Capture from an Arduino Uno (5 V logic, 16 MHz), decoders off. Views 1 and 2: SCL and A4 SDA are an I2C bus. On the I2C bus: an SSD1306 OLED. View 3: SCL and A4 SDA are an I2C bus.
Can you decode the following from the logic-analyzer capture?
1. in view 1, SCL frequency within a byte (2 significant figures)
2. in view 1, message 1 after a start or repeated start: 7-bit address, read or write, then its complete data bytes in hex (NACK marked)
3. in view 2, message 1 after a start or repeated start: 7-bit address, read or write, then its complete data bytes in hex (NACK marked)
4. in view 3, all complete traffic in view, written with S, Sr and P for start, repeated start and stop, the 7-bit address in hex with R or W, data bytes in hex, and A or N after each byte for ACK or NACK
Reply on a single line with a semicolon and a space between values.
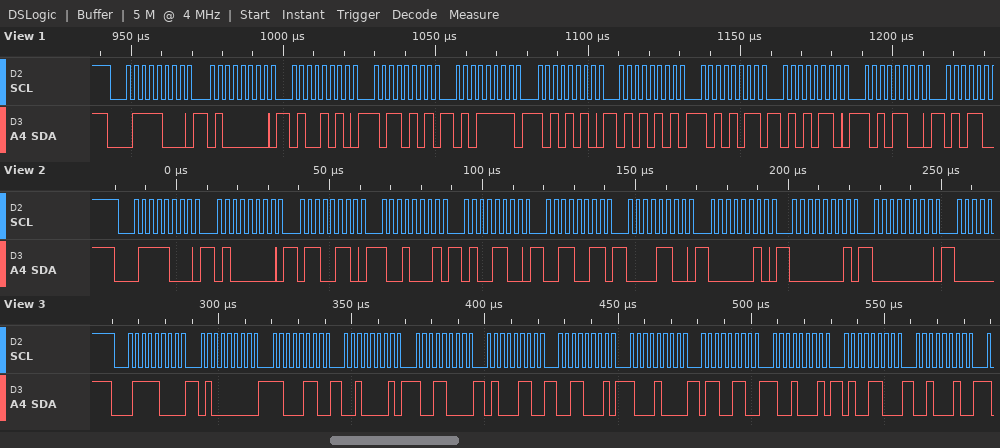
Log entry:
400 kHz; 0x3C write: 40 4A B5 5F AA 55 AB 56 AC; 0x3C write: 40 66 91 4C 33 0C 02 01 00; S 3CW A 40 A C6 A 21 A 98 A 46 A 31 A 88 A 66 A 91 A 4C A 22 A
